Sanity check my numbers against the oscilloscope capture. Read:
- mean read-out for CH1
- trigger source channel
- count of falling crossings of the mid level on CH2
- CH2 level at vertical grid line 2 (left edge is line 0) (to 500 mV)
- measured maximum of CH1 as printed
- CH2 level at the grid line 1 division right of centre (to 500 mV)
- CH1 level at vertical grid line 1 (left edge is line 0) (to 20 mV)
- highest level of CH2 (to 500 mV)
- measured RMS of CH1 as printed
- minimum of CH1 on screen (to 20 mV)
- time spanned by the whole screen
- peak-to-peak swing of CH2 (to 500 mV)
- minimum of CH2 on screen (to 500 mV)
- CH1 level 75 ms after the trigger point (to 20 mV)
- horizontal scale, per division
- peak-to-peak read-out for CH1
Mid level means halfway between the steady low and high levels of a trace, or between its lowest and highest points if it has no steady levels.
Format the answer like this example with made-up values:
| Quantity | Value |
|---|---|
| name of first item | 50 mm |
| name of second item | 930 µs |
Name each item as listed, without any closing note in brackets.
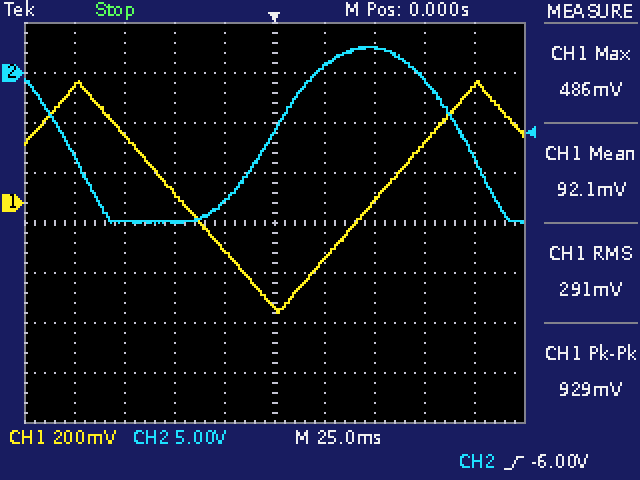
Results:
| Quantity | Value |
|---|---|
| mean read-out for CH1 | 92.1 mV |
| trigger source channel | CH2 |
| count of falling crossings of the mid level on CH2 | 2 |
| CH2 level at vertical grid line 2 (left edge is line 0) | -15.0 V |
| measured maximum of CH1 as printed | 486 mV |
| CH2 level at the grid line 1 division right of centre | 500 mV |
| CH1 level at vertical grid line 1 (left edge is line 0) | 460 mV |
| highest level of CH2 | 2.5 V |
| measured RMS of CH1 as printed | 291 mV |
| minimum of CH1 on screen | -440 mV |
| time spanned by the whole screen | 250 ms |
| peak-to-peak swing of CH2 | 17.5 V |
| minimum of CH2 on screen | -15.0 V |
| CH1 level 75 ms after the trigger point | 240 mV |
| horizontal scale, per division | 25 ms |
| peak-to-peak read-out for CH1 | 929 mV |
